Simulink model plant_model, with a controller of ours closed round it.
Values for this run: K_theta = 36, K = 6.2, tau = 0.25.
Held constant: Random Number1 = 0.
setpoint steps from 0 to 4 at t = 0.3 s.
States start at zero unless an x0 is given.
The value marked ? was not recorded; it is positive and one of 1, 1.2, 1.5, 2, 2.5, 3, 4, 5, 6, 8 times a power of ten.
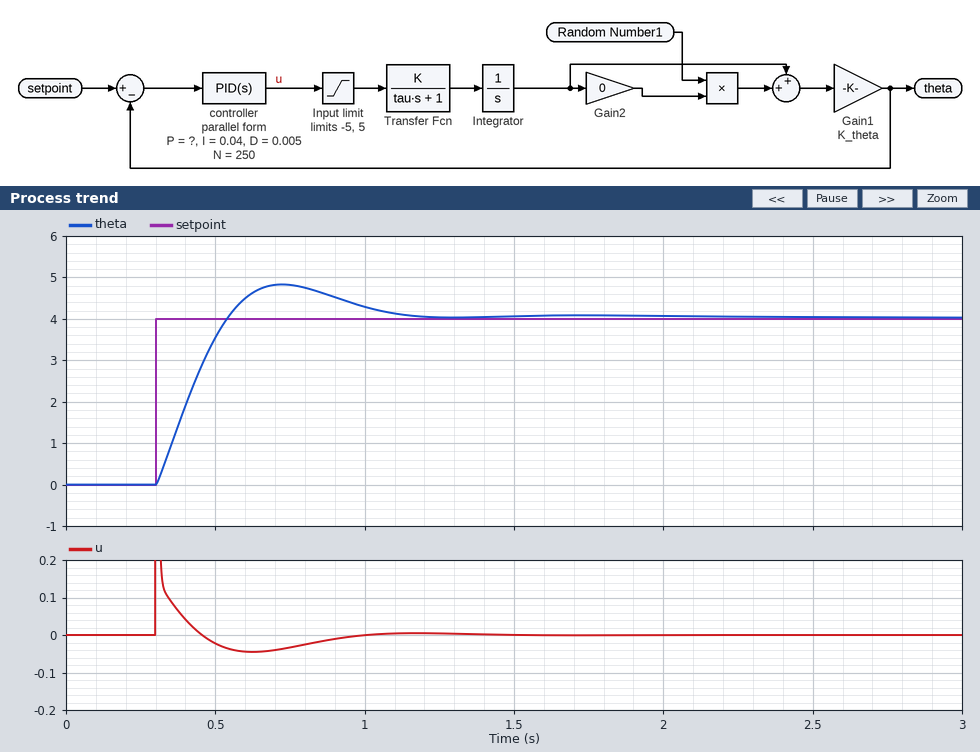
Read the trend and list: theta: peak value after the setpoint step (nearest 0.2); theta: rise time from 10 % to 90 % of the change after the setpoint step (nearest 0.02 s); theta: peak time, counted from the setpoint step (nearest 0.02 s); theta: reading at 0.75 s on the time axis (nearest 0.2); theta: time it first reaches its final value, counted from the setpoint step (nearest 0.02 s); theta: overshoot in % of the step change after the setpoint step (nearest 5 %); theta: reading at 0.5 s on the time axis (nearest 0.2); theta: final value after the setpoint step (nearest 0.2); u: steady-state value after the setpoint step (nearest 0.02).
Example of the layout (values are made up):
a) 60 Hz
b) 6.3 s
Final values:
a) 4.8
b) 0.18 s
c) 0.42 s
d) 4.8
e) 0.24 s
f) 20 %
g) 3.6
h) 4.0
i) 0.00
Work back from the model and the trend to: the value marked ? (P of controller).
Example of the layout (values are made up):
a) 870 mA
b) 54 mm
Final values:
a) 0.06
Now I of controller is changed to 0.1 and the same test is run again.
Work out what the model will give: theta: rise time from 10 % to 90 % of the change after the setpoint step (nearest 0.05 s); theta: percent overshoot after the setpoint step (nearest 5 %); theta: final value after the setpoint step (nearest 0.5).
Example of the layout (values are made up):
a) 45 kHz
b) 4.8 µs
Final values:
a) 0.15 s
b) 30 %
c) 4.0
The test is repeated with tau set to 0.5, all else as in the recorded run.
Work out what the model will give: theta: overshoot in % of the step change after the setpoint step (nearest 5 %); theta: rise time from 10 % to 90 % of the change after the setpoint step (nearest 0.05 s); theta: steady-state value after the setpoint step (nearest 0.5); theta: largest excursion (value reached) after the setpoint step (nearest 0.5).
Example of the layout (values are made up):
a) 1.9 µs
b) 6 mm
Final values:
a) 40 %
b) 0.25 s
c) 4.0
d) 5.5
